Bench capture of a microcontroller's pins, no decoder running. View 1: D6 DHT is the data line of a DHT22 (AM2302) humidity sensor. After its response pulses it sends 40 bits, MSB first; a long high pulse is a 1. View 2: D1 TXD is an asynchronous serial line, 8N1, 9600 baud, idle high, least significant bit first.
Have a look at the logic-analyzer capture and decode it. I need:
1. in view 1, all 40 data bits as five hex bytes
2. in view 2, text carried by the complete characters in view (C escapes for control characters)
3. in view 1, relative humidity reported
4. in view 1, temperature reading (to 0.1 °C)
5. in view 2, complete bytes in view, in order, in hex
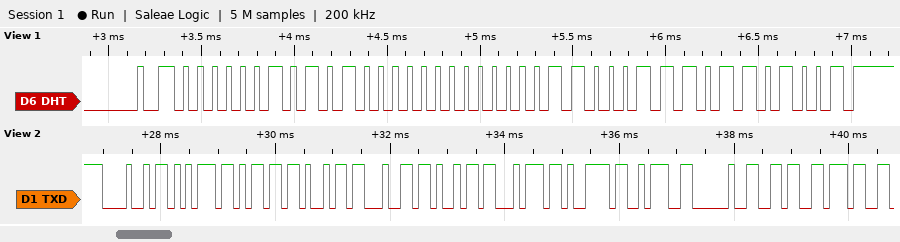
02 A0 00 C7 69
"Humidity: 67"
67.2 %
19.9 °C
48 75 6D 69 64 69 74 79 3A 20 36 37
